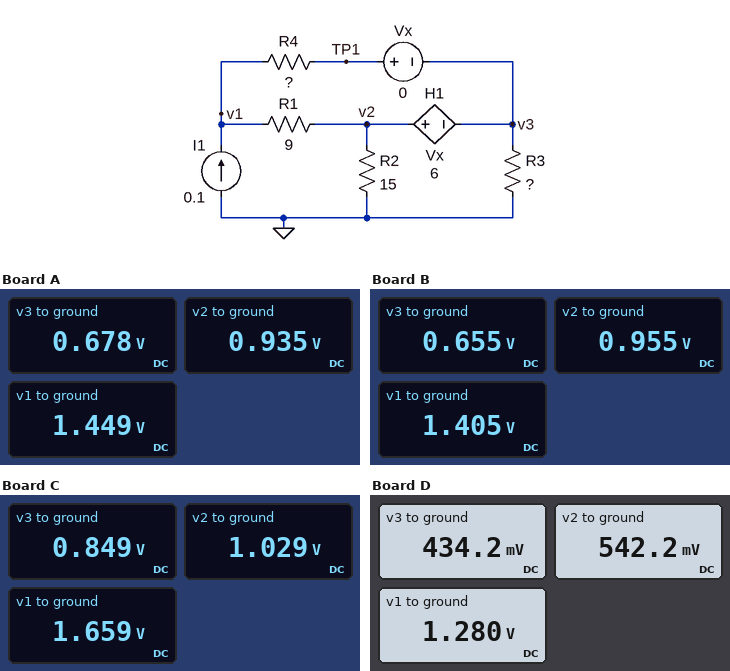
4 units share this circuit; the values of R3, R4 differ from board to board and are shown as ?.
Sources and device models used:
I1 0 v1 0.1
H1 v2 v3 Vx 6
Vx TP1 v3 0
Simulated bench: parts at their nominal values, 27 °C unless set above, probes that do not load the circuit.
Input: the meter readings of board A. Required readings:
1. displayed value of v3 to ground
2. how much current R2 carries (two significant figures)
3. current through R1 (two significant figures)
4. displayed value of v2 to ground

0.678 V
62 mA
57 mA
0.935 V
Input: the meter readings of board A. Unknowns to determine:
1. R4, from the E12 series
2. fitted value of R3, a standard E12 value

18 Ω
18 Ω
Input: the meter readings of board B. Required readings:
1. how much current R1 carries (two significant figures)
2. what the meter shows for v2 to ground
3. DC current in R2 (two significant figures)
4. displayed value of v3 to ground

50 mA
0.955 V
64 mA
0.655 V
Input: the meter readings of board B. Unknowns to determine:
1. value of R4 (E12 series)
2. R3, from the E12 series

15 Ω
18 Ω
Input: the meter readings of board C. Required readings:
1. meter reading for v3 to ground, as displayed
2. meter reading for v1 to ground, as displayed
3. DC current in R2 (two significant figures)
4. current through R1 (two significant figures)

0.849 V
1.659 V
69 mA
70 mA
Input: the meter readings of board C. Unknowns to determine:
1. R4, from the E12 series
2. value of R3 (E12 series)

27 Ω
27 Ω
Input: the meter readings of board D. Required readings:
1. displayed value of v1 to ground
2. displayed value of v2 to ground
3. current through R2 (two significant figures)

1.280 V
542.2 mV
36 mA
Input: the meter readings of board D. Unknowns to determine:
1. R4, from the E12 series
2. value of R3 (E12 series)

47 Ω
6.8 Ω
